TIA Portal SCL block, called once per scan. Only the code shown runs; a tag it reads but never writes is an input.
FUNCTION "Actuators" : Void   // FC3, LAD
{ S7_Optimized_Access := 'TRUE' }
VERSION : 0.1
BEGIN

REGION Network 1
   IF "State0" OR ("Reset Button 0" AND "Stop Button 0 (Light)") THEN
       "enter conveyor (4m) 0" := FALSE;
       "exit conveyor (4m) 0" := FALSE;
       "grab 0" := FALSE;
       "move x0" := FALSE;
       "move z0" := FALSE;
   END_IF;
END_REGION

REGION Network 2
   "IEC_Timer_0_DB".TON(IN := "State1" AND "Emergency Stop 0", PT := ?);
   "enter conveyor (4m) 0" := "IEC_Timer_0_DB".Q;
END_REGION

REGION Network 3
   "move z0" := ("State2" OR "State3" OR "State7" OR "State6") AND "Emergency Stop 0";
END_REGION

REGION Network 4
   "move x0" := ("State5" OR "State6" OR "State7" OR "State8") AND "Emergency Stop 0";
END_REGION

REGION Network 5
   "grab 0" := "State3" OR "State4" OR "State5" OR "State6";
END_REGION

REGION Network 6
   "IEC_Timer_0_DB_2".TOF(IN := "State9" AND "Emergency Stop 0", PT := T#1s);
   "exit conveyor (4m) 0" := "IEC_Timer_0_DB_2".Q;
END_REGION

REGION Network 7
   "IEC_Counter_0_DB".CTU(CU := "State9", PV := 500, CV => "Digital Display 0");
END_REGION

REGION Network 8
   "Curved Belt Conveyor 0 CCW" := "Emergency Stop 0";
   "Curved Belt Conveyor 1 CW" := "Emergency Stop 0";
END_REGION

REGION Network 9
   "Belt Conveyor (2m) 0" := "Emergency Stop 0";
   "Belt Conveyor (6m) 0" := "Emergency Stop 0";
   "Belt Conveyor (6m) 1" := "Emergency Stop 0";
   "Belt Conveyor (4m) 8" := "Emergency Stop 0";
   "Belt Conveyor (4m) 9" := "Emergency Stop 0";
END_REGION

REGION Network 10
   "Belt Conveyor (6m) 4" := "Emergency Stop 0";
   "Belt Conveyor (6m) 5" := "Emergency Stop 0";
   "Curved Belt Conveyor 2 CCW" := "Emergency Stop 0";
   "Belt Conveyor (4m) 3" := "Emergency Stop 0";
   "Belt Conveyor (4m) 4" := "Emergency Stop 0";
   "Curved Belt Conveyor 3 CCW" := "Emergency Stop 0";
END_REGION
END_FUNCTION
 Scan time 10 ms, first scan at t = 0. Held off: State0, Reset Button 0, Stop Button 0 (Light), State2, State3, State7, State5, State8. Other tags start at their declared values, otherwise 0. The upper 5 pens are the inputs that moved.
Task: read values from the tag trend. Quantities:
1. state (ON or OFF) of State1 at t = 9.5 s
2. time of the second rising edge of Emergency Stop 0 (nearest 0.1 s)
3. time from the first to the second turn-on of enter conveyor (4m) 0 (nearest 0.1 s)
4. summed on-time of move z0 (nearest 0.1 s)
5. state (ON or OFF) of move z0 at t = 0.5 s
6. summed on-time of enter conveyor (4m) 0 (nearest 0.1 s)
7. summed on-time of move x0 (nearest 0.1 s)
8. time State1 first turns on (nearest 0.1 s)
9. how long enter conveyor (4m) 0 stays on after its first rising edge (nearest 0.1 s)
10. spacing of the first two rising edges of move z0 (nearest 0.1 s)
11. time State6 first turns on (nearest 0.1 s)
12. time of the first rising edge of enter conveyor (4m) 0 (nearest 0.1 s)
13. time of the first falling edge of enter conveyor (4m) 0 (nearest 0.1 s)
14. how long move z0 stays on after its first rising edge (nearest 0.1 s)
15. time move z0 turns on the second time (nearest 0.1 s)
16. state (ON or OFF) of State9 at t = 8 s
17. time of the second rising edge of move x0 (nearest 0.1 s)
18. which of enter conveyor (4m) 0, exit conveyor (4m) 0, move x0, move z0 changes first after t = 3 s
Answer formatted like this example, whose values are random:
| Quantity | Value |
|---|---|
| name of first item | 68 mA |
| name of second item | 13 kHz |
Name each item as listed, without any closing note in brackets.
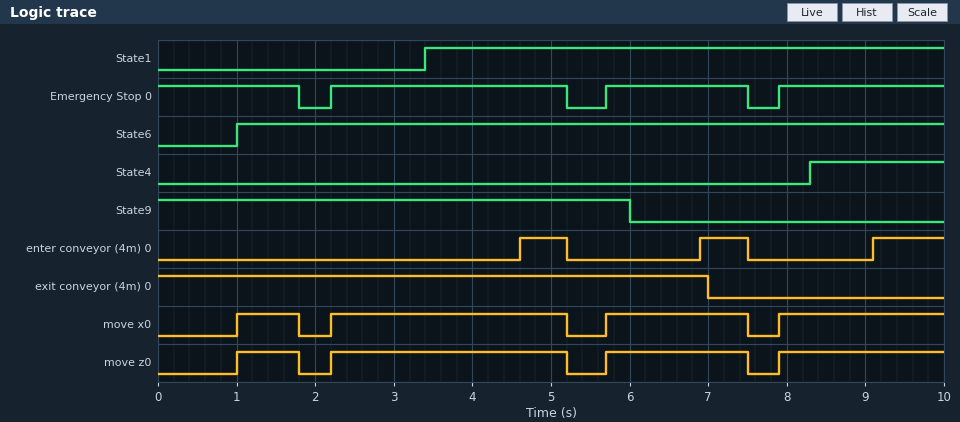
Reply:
| Quantity | Value |
|---|---|
| state (ON or OFF) of State1 at t = 9.5 s | ON |
| time of the second rising edge of Emergency Stop 0 | 5.7 s |
| time from the first to the second turn-on of enter conveyor (4m) 0 | 2.3 s |
| summed on-time of move z0 | 7.7 s |
| state (ON or OFF) of move z0 at t = 0.5 s | OFF |
| summed on-time of enter conveyor (4m) 0 | 2.1 s |
| summed on-time of move x0 | 7.7 s |
| time State1 first turns on | 3.4 s |
| how long enter conveyor (4m) 0 stays on after its first rising edge | 0.6 s |
| spacing of the first two rising edges of move z0 | 1.2 s |
| time State6 first turns on | 1.0 s |
| time of the first rising edge of enter conveyor (4m) 0 | 4.6 s |
| time of the first falling edge of enter conveyor (4m) 0 | 5.2 s |
| how long move z0 stays on after its first rising edge | 0.8 s |
| time move z0 turns on the second time | 2.2 s |
| state (ON or OFF) of State9 at t = 8 s | OFF |
| time of the second rising edge of move x0 | 2.2 s |
| which of enter conveyor (4m) 0, exit conveyor (4m) 0, move x0, move z0 changes first after t = 3 s | enter conveyor (4m) 0 |
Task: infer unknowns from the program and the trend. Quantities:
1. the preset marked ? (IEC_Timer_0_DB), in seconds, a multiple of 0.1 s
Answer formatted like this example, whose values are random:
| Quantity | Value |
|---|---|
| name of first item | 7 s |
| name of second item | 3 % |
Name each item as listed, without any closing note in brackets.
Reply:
| Quantity | Value |
|---|---|
| the preset marked ? (IEC_Timer_0_DB), in seconds, a multiple of 0.1 s | 1.2 s |
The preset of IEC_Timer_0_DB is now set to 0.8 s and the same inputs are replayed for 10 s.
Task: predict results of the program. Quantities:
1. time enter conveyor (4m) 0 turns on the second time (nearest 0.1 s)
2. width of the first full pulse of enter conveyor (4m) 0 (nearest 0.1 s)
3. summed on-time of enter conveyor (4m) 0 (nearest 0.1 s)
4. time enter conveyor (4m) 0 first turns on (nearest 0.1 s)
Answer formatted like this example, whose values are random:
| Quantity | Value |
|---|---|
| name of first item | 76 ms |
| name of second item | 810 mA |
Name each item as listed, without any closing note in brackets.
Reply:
| Quantity | Value |
|---|---|
| time enter conveyor (4m) 0 turns on the second time | 6.5 s |
| width of the first full pulse of enter conveyor (4m) 0 | 1.0 s |
| summed on-time of enter conveyor (4m) 0 | 3.3 s |
| time enter conveyor (4m) 0 first turns on | 4.2 s |
